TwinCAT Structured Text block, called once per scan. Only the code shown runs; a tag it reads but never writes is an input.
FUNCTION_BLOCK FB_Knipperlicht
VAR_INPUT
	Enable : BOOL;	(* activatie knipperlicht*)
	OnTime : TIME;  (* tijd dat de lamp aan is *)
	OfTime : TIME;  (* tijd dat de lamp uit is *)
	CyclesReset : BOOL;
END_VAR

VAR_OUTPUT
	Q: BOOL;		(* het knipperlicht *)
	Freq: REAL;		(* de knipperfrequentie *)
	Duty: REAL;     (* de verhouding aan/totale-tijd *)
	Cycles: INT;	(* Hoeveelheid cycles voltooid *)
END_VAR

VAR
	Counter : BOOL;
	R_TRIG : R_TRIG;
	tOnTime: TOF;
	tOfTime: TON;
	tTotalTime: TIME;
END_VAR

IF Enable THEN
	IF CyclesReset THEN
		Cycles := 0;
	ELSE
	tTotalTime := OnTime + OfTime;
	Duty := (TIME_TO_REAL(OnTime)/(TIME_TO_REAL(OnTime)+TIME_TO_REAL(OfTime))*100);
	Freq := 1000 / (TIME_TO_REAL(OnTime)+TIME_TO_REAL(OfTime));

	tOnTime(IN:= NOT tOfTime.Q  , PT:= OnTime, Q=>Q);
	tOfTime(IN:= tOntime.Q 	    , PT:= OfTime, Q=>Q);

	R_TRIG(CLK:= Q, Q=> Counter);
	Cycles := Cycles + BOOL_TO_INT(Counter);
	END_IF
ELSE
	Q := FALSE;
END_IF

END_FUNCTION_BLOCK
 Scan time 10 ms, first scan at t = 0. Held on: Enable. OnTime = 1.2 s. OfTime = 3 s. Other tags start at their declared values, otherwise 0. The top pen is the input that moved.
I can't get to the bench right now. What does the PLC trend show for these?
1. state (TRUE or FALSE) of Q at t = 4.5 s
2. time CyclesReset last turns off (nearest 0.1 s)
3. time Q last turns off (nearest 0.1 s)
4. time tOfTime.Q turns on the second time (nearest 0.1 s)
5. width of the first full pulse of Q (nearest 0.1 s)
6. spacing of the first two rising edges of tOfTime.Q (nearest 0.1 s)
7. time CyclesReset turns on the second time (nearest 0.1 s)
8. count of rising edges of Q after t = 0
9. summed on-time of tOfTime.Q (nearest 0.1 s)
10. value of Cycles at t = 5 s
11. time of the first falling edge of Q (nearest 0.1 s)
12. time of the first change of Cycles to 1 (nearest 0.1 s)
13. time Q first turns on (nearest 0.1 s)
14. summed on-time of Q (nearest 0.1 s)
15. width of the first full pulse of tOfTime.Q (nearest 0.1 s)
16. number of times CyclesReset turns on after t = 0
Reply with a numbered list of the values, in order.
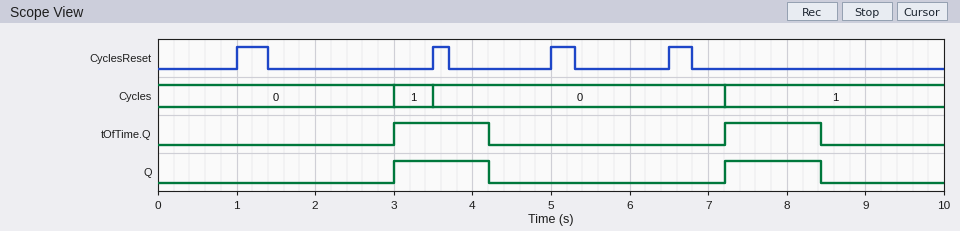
1. FALSE
2. 6.8 s
3. 8.4 s
4. 7.2 s
5. 1.2 s
6. 4.2 s
7. 3.5 s
8. 2
9. 2.4 s
10. 0
11. 4.2 s
12. 3.0 s
13. 3.0 s
14. 2.4 s
15. 1.2 s
16. 4
